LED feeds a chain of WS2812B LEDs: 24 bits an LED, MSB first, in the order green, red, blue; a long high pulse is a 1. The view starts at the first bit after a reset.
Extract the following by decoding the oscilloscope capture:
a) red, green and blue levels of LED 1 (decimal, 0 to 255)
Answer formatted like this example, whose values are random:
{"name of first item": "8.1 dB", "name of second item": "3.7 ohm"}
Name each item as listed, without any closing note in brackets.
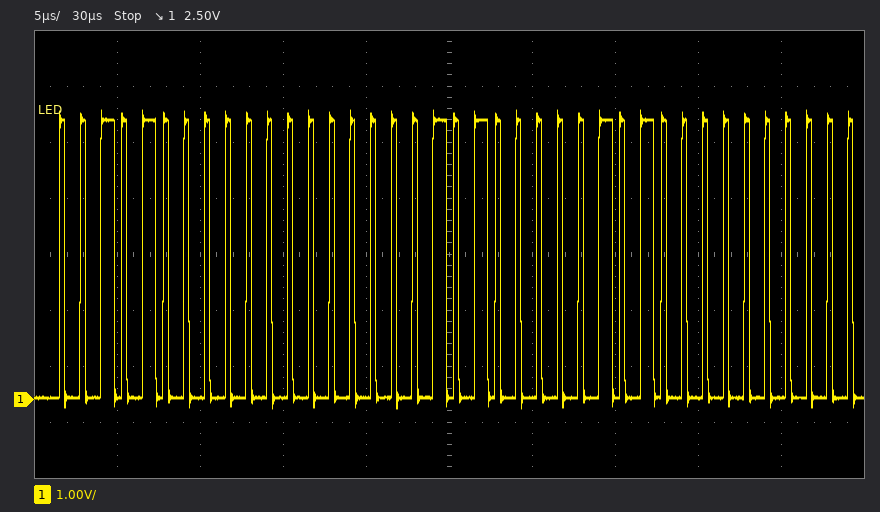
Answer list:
{"red, green and blue levels of LED 1": "0, 40, 40"}
